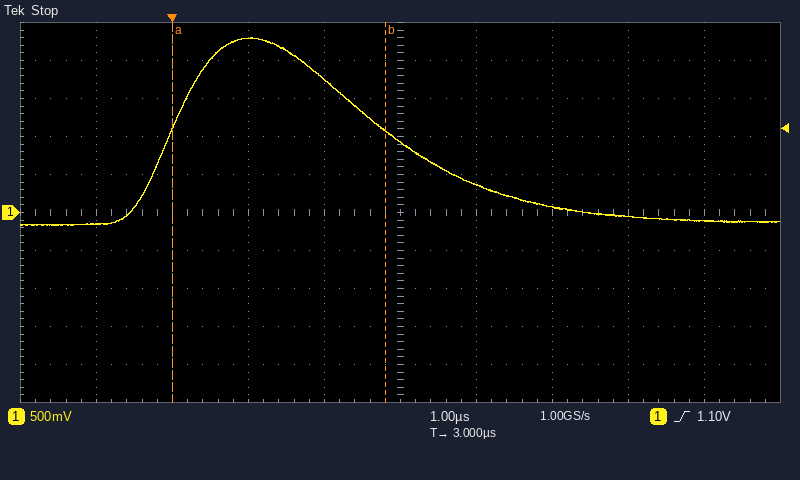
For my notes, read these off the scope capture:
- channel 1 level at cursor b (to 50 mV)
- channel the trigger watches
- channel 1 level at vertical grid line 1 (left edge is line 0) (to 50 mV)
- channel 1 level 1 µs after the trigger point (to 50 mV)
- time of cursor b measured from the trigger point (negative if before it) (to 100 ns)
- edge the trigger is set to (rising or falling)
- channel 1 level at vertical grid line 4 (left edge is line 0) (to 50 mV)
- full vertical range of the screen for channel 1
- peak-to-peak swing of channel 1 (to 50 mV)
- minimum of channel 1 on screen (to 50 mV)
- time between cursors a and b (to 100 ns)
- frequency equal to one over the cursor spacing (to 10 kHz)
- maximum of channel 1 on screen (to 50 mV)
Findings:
1.05 V
channel 1
-150 mV
2.30 V
+2.8 µs
rising
1.75 V
5 V
2.45 V
-150 mV
2.8 µs
360 kHz
2.30 V
